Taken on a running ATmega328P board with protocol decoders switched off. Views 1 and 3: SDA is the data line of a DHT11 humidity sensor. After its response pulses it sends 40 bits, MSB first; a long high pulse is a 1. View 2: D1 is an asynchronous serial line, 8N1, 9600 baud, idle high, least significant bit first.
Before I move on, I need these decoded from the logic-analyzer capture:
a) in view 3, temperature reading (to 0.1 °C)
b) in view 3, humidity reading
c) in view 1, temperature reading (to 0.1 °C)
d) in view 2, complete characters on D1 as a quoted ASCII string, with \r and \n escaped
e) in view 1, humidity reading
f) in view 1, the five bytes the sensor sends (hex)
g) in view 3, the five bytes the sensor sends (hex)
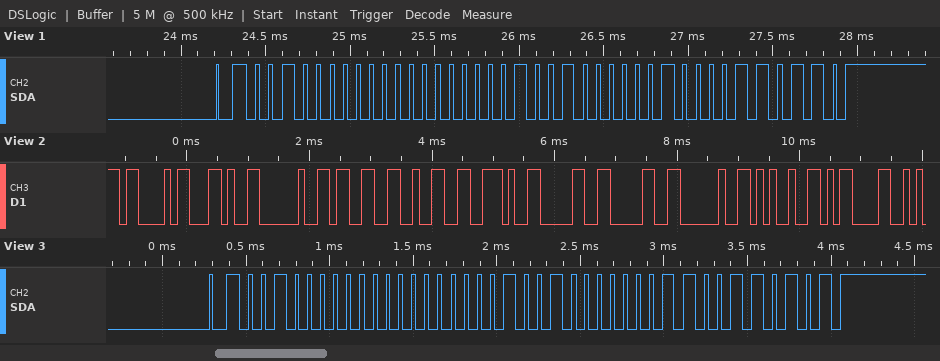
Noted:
18.3 °C
32 %
18.4 °C
"C, 32.00 %\r"
32 %
20 00 12 04 36
20 00 12 03 35
